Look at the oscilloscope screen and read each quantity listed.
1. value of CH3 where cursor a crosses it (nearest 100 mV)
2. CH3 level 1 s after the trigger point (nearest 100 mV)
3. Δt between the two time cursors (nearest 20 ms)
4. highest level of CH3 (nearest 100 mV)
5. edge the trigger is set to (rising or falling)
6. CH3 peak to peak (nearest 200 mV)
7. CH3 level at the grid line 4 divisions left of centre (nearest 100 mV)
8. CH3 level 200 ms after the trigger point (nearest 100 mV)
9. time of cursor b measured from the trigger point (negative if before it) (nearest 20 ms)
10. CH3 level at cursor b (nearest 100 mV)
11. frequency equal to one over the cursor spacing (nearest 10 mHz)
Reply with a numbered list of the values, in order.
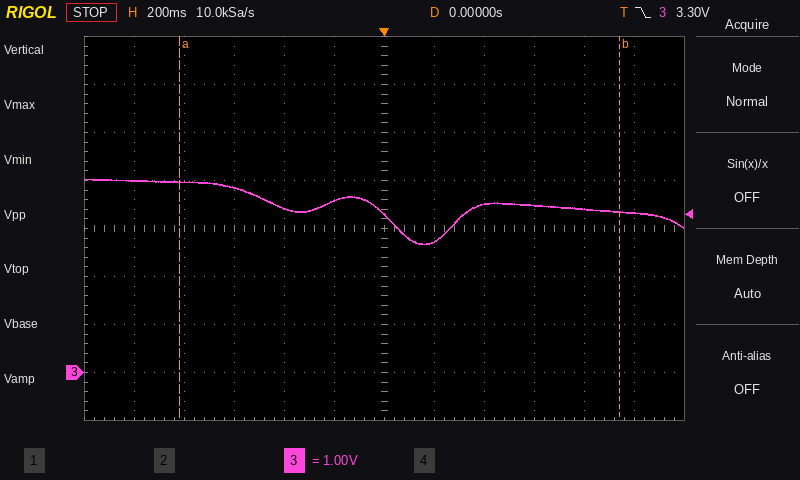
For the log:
1. 4.0 V
2. 3.3 V
3. 1.76 s
4. 4.0 V
5. falling
6. 1.4 V
7. 4.0 V
8. 2.7 V
9. +940 ms
10. 3.3 V
11. 570 mHz
